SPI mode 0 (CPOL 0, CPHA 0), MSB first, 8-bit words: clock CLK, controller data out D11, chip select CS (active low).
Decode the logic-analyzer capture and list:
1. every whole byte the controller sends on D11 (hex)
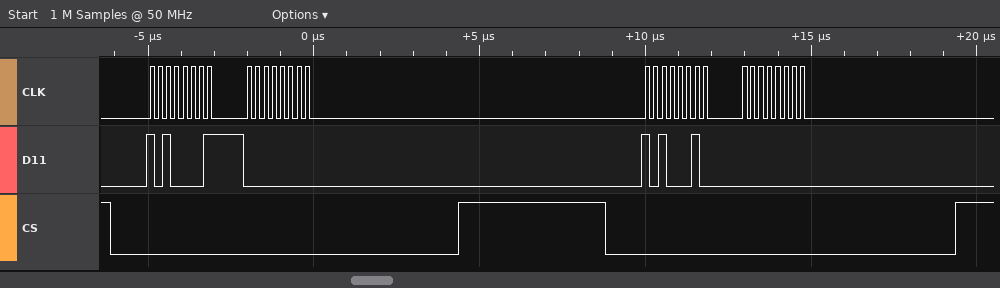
A1 00 A2 00
